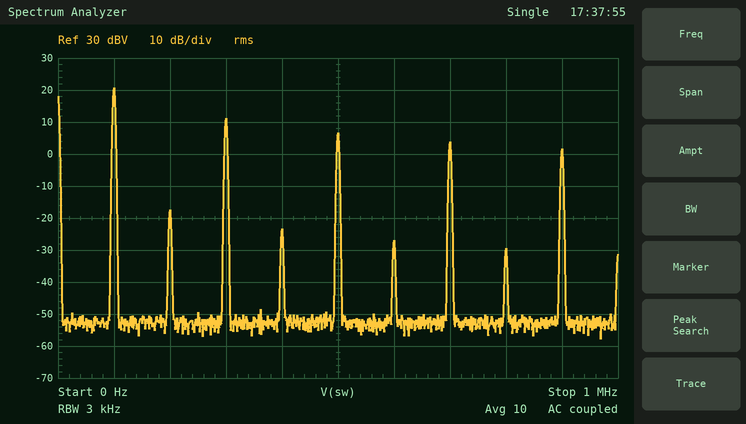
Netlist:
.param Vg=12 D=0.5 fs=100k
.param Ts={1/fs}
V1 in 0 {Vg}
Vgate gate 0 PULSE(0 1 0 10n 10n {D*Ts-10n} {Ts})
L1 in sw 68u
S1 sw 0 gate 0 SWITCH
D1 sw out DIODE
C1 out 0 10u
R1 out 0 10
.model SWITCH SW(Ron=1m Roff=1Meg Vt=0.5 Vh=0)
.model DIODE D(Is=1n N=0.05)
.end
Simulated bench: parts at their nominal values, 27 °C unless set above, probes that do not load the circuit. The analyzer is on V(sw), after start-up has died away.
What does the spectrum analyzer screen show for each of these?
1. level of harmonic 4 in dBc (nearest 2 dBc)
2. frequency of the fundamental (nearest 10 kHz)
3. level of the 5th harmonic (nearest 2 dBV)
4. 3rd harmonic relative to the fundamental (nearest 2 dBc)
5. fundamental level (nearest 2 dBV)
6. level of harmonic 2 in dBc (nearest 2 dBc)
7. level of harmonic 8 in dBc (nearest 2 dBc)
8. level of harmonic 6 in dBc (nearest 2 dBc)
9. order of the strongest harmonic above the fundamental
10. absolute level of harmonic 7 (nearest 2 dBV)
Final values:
-44 dBc
100 kHz
6 dBV
-10 dBc
20 dBV
-38 dBc
-50 dBc
-48 dBc
3
4 dBV
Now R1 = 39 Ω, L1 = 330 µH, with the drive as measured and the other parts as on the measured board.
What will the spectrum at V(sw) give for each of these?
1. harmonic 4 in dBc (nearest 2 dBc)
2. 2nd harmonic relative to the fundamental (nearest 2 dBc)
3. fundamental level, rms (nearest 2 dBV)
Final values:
-56 dBc
-50 dBc
20 dBV
